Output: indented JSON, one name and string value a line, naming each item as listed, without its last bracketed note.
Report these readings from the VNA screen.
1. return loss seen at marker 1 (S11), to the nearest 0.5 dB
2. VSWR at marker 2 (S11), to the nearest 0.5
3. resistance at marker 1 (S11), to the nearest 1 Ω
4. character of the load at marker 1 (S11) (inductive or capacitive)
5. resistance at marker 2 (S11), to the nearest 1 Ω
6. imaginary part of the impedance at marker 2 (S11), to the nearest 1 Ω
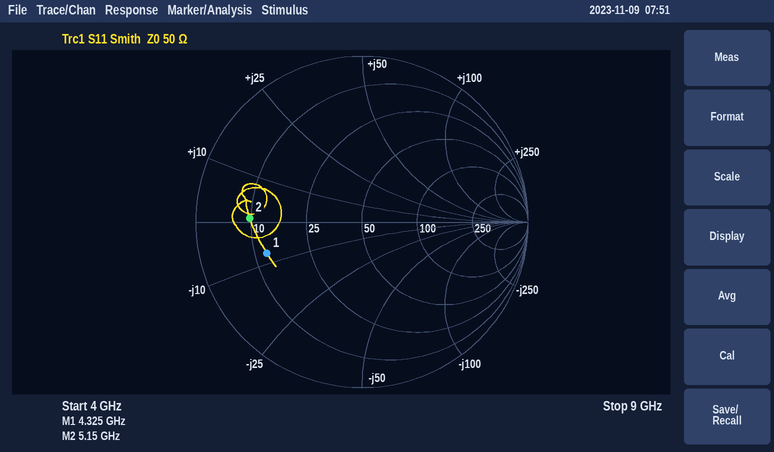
{
  "return loss seen at marker 1 (S11), to the nearest 0.5 dB": "4.5 dB",
  "VSWR at marker 2 (S11), to the nearest 0.5": "5.0",
  "resistance at marker 1 (S11), to the nearest 1 Ω": "13 Ω",
  "character of the load at marker 1 (S11)": "capacitive",
  "resistance at marker 2 (S11), to the nearest 1 Ω": "10 Ω",
  "imaginary part of the impedance at marker 2 (S11), to the nearest 1 Ω": "+1 Ω"
}
